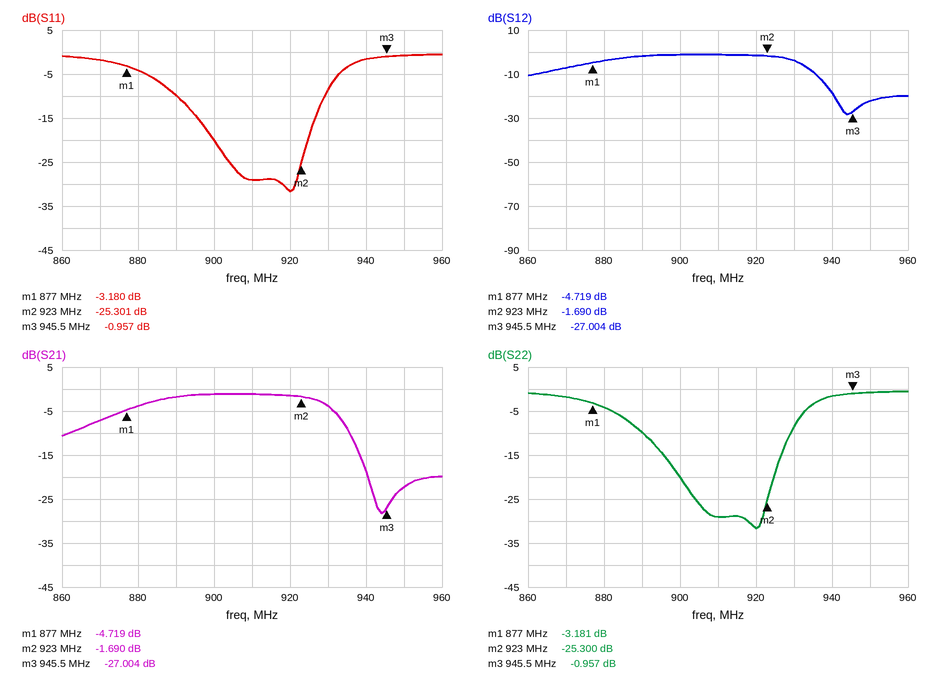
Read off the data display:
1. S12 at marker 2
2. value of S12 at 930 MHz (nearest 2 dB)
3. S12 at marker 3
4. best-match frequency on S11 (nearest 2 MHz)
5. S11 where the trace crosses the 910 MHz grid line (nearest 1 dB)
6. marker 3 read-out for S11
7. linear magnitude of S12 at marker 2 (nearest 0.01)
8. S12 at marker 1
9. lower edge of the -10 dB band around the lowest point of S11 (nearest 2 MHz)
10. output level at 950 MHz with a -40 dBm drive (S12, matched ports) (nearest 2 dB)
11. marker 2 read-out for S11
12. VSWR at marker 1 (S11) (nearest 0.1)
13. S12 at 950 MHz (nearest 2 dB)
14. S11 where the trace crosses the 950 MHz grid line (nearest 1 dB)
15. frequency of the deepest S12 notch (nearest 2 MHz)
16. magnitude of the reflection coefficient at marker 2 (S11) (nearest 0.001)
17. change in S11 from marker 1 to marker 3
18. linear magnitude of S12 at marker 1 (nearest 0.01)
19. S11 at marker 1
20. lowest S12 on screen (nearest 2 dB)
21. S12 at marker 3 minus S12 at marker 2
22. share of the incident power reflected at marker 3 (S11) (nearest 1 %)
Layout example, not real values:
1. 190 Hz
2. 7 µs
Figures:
1. -1.690 dB
2. -4 dB
3. -27.004 dB
4. 920 MHz
5. -29 dB
6. -0.957 dB
7. 0.82
8. -4.719 dB
9. 890 MHz
10. -62 dBm
11. -25.301 dB
12. 5.5
13. -22 dB
14. -1 dB
15. 944 MHz
16. 0.054
17. 2.223 dB
18. 0.58
19. -3.180 dB
20. -28 dB
21. -25.314 dB
22. 80 %
